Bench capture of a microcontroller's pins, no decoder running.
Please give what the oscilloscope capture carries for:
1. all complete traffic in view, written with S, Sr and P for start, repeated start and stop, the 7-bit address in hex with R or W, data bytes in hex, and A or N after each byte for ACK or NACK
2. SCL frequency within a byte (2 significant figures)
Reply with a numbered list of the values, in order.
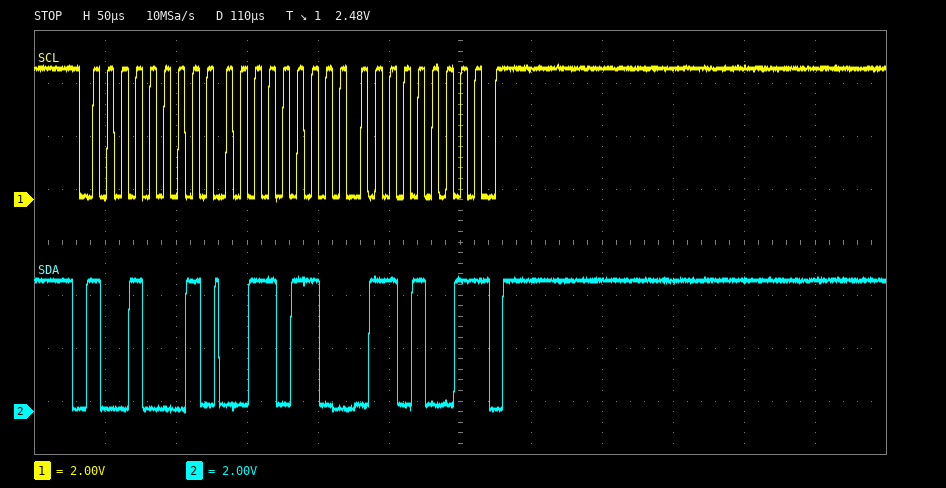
1. S 48R A 36 A 69 N P
2. 100 kHz
